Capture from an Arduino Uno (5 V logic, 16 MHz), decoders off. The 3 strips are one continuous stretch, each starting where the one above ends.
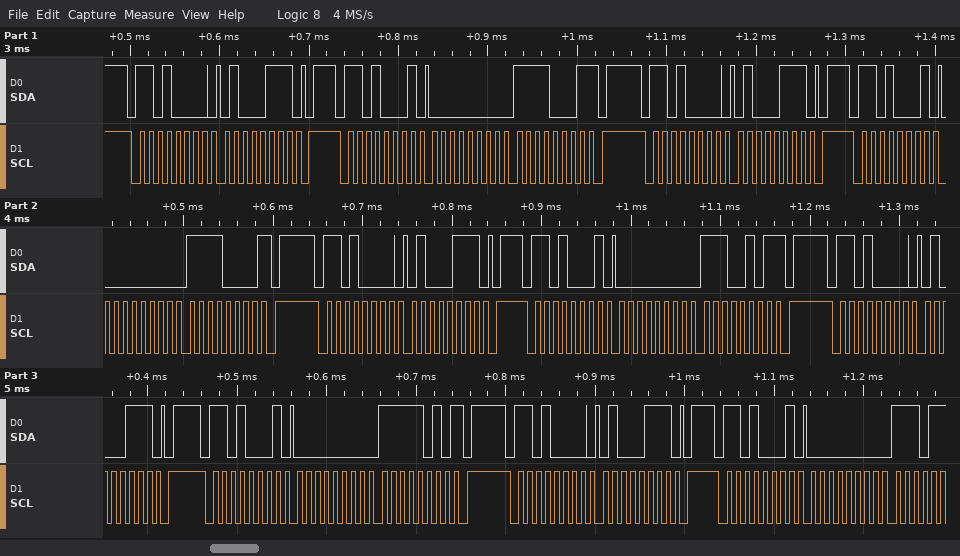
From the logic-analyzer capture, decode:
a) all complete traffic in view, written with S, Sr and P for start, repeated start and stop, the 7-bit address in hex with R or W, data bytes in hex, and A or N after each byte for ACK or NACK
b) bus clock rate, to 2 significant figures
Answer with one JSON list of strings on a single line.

["S 68W A 47 A P S 68R A 00 A F1 N P S 68W A 47 A P S 68R A 00 A F0 N P S 68W A 47 A P S 68R A 00 A E5 N P S 68W A 47 A P S 68R A 00 A FA N P S 68W A 47 A P S 68R A 00 A", "100 kHz"]
